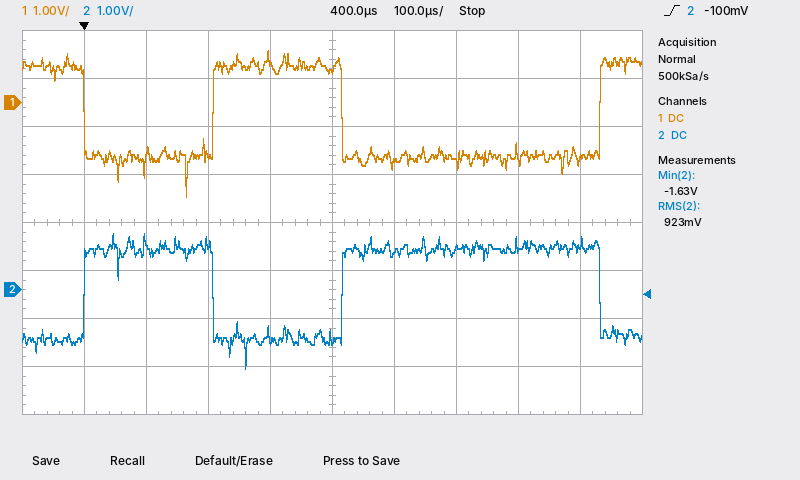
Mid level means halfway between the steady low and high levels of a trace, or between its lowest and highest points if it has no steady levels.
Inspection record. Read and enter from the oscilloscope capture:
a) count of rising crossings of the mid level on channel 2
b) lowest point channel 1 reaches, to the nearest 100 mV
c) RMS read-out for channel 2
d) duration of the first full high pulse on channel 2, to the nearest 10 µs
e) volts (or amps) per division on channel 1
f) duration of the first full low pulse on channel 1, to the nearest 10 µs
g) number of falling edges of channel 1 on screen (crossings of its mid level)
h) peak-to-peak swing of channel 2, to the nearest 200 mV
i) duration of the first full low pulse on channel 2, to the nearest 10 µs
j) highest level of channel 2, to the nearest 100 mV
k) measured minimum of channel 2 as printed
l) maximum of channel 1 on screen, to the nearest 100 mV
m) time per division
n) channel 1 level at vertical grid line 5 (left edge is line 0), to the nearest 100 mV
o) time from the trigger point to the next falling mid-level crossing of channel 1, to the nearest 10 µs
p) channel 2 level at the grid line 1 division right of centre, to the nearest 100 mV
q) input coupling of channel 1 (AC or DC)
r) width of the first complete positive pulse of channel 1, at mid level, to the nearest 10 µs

2
-2.0 V
923 mV
210 µs
1 V
210 µs
2
2.8 V
210 µs
1.2 V
-1.63 V
1.1 V
100 µs
700 mV
420 µs
800 mV
DC
210 µs
